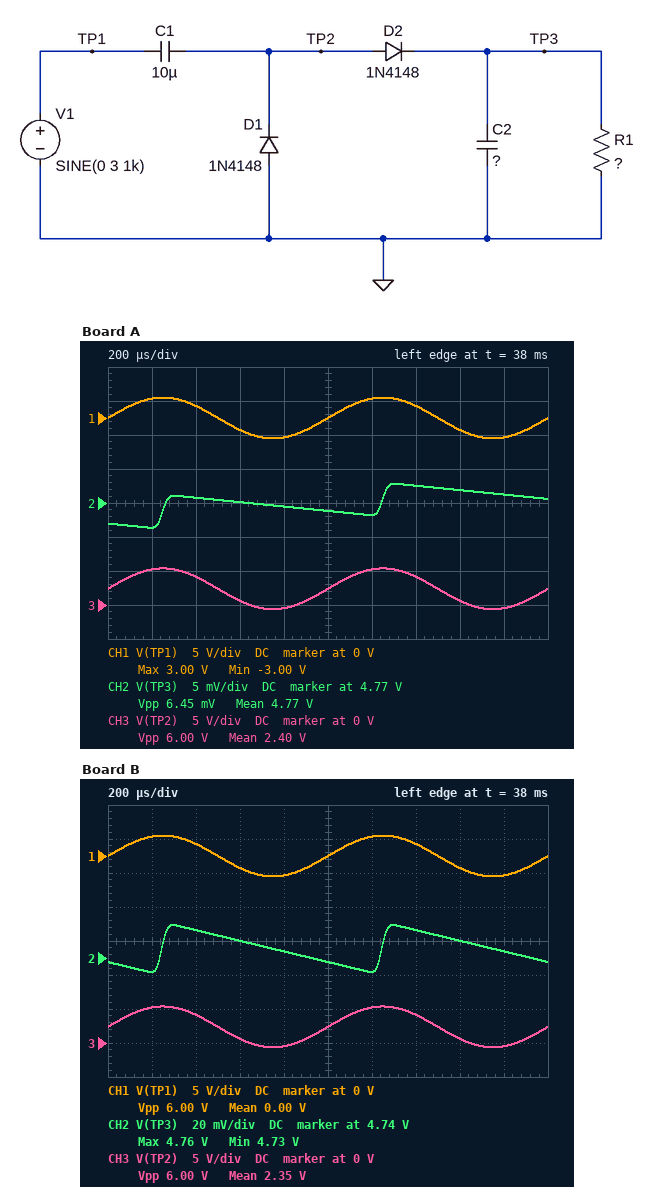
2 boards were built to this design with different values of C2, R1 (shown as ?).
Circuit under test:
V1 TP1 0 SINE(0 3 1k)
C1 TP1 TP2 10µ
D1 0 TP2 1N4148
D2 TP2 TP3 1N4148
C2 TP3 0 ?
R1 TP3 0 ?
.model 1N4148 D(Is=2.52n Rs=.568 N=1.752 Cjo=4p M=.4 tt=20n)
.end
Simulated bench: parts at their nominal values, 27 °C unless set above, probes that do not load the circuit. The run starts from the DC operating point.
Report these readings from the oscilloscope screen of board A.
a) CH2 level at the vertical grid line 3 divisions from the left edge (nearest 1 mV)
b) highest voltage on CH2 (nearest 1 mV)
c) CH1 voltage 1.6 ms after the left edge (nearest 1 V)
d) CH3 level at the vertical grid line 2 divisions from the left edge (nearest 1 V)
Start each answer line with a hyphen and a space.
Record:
- 4.770 V
- 4.773 V
- -2 V
- 4 V
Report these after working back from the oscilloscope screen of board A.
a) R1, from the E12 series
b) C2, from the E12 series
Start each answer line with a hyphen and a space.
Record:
- 82 kΩ
- 18 µF
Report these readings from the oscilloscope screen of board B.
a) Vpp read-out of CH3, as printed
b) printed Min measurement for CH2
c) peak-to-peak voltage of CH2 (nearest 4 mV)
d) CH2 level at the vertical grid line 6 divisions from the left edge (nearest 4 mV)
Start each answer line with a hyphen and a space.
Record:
- 6.00 V
- 4.73 V
- 28 mV
- 4.732 V
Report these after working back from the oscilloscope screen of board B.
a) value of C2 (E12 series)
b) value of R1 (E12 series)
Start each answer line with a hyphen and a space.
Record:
- 3.9 µF
- 39 kΩ
